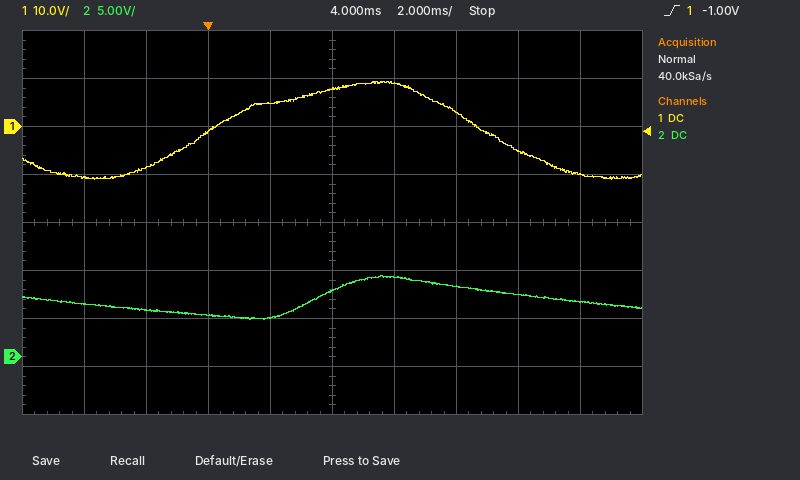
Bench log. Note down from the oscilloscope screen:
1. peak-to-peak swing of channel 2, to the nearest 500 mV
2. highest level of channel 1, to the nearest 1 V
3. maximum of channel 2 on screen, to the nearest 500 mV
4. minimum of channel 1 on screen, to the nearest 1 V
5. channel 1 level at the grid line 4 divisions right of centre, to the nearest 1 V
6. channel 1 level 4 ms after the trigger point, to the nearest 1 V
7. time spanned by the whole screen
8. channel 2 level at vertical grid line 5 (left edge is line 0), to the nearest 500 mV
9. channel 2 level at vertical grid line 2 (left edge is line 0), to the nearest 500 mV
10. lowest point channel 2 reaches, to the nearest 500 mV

4.5 V
9 V
8.5 V
-11 V
-10 V
8 V
20 ms
7.0 V
5.0 V
4.0 V
